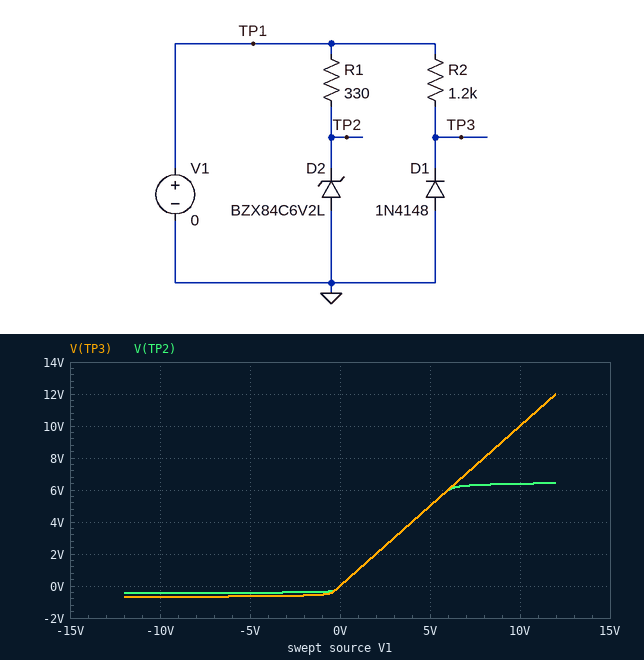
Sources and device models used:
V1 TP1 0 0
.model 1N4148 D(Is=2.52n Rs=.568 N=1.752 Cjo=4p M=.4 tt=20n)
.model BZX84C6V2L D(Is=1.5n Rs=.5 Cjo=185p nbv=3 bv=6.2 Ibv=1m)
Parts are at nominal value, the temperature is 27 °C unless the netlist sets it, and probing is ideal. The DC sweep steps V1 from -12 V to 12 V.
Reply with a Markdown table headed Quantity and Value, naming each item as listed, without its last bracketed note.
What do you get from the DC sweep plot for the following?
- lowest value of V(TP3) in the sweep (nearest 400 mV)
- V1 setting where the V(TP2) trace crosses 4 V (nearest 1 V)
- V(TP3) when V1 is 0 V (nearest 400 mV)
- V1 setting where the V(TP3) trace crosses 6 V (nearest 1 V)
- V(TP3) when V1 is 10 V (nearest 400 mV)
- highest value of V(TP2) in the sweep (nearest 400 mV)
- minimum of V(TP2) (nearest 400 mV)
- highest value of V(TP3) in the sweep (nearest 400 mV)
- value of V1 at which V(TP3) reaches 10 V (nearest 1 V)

| Quantity | Value |
|---|---|
| lowest value of V(TP3) in the sweep | -800 mV |
| V1 setting where the V(TP2) trace crosses 4 V | 4 V |
| V(TP3) when V1 is 0 V | 0 V |
| V1 setting where the V(TP3) trace crosses 6 V | 6 V |
| V(TP3) when V1 is 10 V | 10.0 V |
| highest value of V(TP2) in the sweep | 6.4 V |
| minimum of V(TP2) | -400 mV |
| highest value of V(TP3) in the sweep | 12.0 V |
| value of V1 at which V(TP3) reaches 10 V | 10 V |
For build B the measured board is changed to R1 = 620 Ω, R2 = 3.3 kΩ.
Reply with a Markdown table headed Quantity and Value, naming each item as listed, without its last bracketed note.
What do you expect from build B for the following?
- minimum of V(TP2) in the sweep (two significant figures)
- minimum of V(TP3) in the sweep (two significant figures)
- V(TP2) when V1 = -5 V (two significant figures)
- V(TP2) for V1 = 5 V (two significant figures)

| Quantity | Value |
|---|---|
| minimum of V(TP2) in the sweep | -430 mV |
| minimum of V(TP3) in the sweep | -640 mV |
| V(TP2) when V1 = -5 V | -400 mV |
| V(TP2) for V1 = 5 V | 5.0 V |
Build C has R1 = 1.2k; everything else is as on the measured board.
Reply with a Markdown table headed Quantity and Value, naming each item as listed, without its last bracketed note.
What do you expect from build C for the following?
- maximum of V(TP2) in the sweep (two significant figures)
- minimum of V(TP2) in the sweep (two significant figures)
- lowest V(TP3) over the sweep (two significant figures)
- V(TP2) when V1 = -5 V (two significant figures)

| Quantity | Value |
|---|---|
| maximum of V(TP2) in the sweep | 6.3 V |
| minimum of V(TP2) in the sweep | -410 mV |
| lowest V(TP3) over the sweep | -690 mV |
| V(TP2) when V1 = -5 V | -380 mV |
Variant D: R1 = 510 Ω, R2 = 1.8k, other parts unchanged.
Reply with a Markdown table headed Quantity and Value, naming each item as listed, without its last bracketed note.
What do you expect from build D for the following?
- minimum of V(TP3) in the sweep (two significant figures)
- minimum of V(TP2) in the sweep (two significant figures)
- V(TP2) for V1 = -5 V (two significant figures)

| Quantity | Value |
|---|---|
| minimum of V(TP3) in the sweep | -670 mV |
| minimum of V(TP2) in the sweep | -440 mV |
| V(TP2) for V1 = -5 V | -410 mV |
